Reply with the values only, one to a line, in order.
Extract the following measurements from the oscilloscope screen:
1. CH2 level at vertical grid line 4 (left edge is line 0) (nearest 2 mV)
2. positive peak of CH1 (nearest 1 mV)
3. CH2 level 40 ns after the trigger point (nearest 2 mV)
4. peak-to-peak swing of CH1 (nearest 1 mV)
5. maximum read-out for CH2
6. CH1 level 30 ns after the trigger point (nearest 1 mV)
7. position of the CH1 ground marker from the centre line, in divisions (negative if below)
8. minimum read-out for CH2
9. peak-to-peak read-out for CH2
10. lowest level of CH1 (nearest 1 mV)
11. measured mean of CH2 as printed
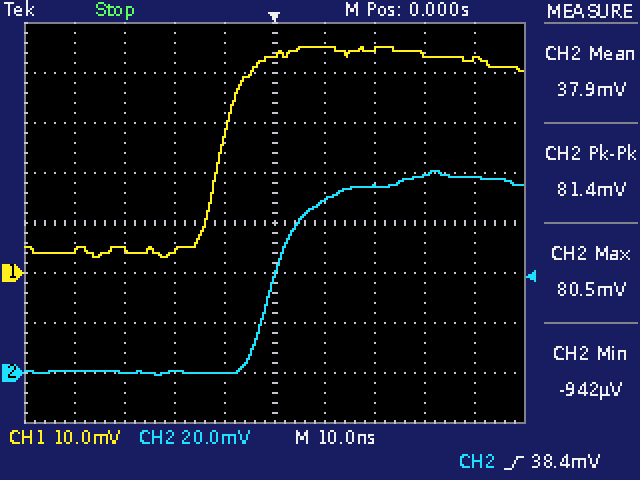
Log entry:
0 mV
45 mV
78 mV
42 mV
80.5 mV
44 mV
-1.0 div
-942 µV
81.4 mV
3 mV
37.9 mV
